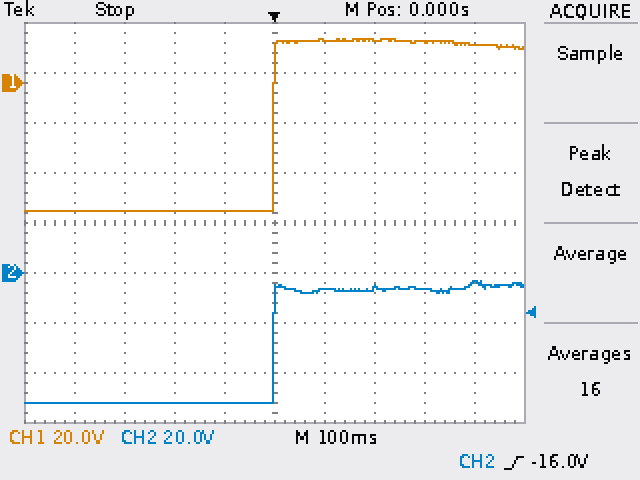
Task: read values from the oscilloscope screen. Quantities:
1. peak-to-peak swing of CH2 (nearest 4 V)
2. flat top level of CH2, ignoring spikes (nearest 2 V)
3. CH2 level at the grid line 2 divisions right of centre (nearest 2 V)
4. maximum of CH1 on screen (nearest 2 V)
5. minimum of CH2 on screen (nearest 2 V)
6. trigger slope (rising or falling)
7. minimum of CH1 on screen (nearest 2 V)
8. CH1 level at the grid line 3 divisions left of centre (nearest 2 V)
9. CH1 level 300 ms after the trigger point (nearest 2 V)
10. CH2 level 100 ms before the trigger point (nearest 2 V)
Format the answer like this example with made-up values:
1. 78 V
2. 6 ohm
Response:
1. 48 V
2. -6 V
3. -6 V
4. 18 V
5. -52 V
6. rising
7. -52 V
8. -52 V
9. 16 V
10. -52 V
